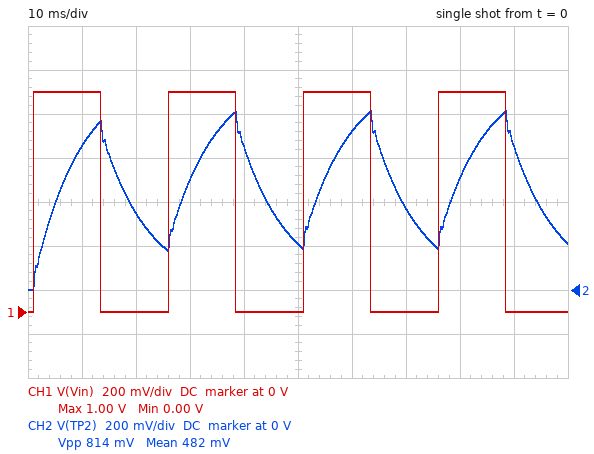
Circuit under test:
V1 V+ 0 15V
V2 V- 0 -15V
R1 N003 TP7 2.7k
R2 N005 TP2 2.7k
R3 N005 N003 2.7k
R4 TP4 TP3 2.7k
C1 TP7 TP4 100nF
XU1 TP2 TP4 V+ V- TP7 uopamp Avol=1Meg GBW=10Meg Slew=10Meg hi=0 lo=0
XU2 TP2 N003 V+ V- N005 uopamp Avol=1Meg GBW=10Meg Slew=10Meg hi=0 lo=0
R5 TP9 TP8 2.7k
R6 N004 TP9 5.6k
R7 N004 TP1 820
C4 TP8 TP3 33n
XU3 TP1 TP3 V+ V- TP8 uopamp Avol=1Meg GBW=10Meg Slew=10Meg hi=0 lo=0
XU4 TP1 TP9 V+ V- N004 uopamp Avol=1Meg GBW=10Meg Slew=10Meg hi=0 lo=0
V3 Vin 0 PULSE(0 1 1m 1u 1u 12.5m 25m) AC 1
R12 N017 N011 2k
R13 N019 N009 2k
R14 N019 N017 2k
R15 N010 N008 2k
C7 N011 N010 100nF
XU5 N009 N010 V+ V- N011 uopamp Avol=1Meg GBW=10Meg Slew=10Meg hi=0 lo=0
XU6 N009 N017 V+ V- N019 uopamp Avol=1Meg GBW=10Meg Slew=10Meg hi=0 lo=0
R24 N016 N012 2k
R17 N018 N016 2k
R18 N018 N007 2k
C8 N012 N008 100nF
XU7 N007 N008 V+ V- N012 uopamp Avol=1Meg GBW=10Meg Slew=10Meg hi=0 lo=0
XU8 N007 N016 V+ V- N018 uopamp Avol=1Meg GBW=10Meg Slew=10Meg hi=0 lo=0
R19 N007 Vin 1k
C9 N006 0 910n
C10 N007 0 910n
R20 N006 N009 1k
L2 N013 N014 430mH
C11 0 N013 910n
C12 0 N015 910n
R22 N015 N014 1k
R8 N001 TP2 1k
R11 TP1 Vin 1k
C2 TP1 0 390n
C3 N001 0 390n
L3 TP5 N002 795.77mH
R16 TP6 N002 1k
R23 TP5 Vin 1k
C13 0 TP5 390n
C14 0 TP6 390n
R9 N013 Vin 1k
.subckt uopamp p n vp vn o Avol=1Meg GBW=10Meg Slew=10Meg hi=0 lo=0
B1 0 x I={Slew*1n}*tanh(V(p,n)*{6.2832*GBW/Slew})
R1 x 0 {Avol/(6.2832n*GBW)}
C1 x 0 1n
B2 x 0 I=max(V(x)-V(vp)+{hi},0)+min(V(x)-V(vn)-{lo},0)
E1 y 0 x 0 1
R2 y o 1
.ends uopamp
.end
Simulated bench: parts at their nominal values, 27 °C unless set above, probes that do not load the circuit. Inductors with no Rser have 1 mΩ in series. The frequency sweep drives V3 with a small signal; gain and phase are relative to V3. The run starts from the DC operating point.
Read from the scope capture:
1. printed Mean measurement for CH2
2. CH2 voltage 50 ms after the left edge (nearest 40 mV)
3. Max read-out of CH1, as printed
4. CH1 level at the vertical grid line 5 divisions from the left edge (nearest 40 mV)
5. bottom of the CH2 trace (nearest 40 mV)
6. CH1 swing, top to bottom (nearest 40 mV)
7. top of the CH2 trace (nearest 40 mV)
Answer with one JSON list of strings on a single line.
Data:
["482 mV", "200 mV", "1.00 V", "0 V", "0 V", "1.00 V", "800 mV"]
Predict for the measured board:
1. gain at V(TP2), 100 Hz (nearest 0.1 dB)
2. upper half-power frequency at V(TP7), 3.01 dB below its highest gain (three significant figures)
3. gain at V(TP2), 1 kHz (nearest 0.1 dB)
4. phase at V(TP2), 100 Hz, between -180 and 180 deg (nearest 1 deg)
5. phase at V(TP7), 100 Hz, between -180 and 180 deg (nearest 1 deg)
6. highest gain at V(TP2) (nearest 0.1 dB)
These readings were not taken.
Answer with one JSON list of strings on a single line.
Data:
["-14.7 dB", "18.2 Hz", "-21.8 dB", "-68 deg", "-104 deg", "0 dB"]
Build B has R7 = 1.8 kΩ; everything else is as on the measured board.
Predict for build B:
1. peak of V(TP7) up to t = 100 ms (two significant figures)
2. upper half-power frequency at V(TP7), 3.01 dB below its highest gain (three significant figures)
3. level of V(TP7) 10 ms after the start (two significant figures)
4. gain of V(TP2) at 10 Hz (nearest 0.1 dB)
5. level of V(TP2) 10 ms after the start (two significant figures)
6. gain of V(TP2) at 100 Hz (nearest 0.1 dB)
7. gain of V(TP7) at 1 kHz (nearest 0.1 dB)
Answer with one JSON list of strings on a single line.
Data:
["1.1 V", "37.4 Hz", "850 mV", "-0.3 dB", "880 mV", "-9.0 dB", "-11.6 dB"]
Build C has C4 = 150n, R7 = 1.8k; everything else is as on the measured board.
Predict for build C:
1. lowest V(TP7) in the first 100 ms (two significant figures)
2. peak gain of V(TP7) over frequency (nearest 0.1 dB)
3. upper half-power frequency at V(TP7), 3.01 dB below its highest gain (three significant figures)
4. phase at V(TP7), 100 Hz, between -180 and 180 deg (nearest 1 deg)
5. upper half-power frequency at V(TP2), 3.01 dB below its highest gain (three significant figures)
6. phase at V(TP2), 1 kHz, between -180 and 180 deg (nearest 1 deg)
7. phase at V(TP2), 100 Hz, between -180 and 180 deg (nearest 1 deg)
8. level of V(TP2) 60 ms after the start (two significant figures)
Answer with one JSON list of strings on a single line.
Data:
["-220 mV", "0 dB", "226 Hz", "-72 deg", "144 Hz", "-159 deg", "-36 deg", "1.0 V"]
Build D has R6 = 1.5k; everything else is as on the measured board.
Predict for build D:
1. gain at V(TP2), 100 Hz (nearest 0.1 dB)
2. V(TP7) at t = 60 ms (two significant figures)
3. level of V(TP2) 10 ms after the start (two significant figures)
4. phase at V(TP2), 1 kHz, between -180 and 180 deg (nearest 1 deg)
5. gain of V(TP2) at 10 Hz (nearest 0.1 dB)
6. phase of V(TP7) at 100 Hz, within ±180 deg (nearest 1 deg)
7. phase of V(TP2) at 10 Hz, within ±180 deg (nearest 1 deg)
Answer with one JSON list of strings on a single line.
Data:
["-5.8 dB", "950 mV", "960 mV", "-141 deg", "-0.1 dB", "-88 deg", "-9 deg"]
